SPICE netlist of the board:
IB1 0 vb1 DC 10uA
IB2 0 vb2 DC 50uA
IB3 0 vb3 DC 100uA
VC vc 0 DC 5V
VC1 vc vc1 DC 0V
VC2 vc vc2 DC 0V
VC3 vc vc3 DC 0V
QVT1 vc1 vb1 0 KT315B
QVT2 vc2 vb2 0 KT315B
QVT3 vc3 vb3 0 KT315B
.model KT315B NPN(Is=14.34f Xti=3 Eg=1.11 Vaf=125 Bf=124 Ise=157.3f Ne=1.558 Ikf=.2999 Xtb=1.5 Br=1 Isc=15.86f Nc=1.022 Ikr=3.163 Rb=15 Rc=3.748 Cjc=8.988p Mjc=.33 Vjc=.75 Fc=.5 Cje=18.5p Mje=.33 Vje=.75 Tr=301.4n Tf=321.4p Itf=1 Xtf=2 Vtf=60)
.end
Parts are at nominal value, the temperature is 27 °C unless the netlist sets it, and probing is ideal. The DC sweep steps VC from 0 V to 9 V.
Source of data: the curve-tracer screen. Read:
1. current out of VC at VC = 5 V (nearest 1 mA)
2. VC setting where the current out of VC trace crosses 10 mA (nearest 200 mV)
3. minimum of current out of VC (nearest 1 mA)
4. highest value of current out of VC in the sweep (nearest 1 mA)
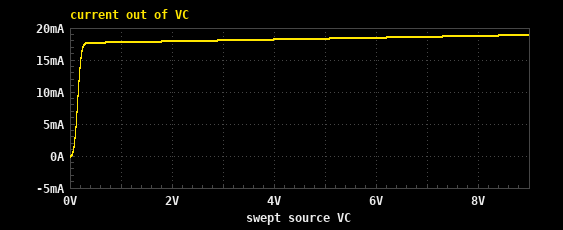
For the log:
18 mA
200 mV
0 A
19 mA
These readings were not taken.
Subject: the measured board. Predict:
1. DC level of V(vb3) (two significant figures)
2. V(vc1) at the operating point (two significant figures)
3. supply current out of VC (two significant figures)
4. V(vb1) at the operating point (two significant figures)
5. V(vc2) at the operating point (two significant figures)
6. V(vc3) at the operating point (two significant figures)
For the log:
710 mV
5.0 V
18 mA
650 mV
5.0 V
5.0 V
